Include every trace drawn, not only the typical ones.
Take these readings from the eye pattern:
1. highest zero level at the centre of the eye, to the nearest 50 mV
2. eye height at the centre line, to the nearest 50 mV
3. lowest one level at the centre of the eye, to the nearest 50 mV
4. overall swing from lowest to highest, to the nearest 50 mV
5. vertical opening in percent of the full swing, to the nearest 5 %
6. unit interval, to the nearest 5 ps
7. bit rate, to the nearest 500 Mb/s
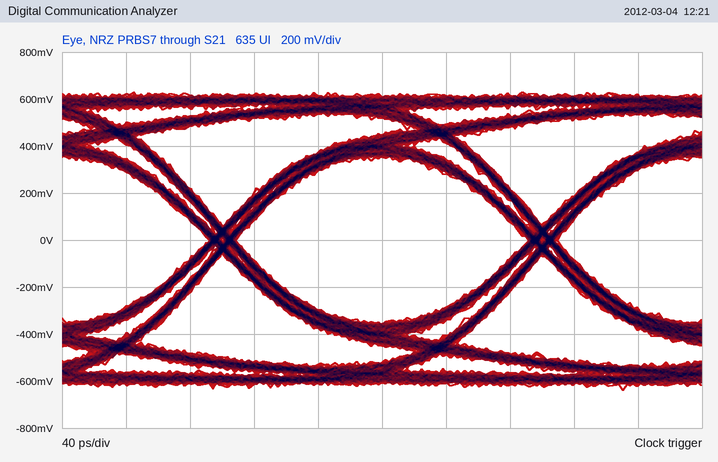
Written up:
-350 mV
700 mV
350 mV
1.25 V
55 %
200 ps
5.0 Gb/s
